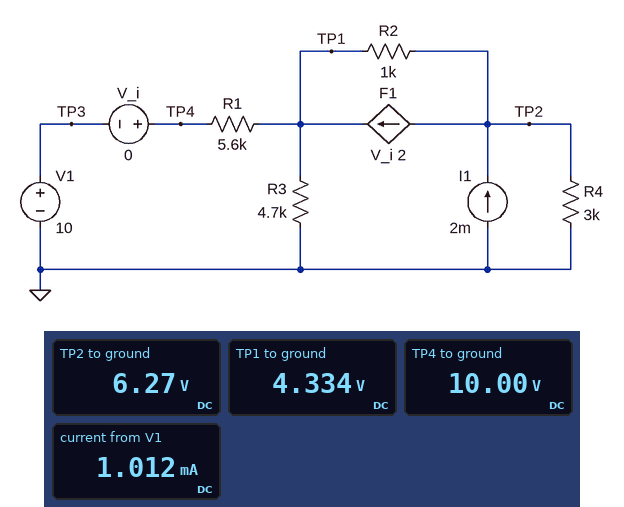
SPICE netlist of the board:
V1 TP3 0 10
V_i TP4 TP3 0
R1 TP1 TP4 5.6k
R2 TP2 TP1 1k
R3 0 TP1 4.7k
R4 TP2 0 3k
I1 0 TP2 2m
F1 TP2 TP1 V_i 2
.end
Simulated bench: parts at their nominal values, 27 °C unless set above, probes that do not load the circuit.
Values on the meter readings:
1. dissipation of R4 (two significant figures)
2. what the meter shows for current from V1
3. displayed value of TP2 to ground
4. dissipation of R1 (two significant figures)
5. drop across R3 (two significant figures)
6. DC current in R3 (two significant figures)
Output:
13 mW
1.012 mA
6.27 V
5.7 mW
4.3 V
920 µA
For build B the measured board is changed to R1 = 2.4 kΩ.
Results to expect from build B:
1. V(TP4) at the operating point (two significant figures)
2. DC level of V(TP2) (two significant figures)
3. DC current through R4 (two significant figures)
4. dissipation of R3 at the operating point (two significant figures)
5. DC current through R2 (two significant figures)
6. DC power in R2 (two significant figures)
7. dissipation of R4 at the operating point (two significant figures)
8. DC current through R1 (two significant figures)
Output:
10 V
8.4 V
2.8 mA
6.1 mW
3.1 mA
9.5 mW
24 mW
1.9 mA
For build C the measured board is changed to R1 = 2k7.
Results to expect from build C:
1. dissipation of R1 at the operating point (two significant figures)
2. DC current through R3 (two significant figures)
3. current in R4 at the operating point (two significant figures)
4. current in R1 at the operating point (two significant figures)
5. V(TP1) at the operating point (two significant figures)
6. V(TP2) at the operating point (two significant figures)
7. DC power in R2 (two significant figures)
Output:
8.6 mW
1.1 mA
2.7 mA
1.8 mA
5.2 V
8.1 V
8.3 mW
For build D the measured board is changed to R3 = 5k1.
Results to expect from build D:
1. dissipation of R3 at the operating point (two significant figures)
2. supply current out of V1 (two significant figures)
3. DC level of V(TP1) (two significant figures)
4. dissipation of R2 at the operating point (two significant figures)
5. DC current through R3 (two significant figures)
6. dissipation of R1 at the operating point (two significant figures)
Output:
3.9 mW
990 µA
4.5 V
3.5 mW
880 µA
5.5 mW
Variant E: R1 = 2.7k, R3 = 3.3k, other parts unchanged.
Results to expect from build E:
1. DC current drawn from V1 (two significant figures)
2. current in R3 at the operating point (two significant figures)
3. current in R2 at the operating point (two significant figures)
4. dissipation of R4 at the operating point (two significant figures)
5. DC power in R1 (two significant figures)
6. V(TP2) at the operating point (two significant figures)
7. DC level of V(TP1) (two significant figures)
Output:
2.0 mA
1.4 mA
3.4 mA
21 mW
11 mW
7.9 V
4.5 V
